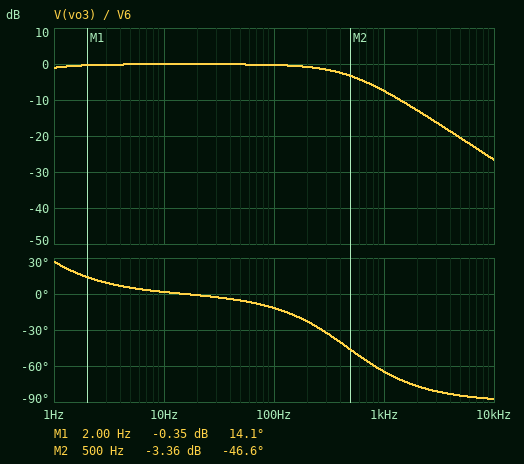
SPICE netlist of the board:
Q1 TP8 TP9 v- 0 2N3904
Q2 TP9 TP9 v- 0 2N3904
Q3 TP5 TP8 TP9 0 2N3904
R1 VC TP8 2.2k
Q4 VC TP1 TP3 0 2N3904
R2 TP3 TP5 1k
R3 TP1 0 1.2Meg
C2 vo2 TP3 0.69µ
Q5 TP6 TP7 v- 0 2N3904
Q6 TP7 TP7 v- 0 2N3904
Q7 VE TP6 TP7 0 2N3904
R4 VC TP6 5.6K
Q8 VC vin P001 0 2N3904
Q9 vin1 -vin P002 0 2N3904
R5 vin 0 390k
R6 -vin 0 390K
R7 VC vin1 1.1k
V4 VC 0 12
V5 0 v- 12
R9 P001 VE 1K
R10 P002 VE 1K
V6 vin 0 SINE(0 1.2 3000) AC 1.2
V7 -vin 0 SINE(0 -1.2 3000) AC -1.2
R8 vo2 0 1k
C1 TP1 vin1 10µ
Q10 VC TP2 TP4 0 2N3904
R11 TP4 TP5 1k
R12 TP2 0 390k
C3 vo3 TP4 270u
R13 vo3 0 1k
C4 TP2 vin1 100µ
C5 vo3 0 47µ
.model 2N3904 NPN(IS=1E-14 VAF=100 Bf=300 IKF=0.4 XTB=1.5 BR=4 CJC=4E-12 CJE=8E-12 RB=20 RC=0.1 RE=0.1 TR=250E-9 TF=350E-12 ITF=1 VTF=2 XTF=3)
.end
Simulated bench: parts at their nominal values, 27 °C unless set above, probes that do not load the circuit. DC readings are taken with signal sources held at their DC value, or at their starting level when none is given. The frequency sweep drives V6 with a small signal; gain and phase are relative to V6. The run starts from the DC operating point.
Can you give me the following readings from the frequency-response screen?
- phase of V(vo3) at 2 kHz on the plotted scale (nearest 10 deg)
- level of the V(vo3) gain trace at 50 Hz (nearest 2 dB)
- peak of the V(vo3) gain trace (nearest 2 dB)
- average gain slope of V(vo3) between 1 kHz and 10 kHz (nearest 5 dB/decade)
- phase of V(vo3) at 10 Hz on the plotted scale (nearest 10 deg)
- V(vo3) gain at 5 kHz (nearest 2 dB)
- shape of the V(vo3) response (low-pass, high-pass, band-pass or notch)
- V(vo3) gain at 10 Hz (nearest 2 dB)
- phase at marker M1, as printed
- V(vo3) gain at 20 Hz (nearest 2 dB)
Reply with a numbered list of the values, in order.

1. -80 deg
2. 0 dB
3. 0 dB
4. -20 dB/decade
5. 0 deg
6. -20 dB
7. low-pass
8. 0 dB
9. 14.1 deg
10. 0 dB
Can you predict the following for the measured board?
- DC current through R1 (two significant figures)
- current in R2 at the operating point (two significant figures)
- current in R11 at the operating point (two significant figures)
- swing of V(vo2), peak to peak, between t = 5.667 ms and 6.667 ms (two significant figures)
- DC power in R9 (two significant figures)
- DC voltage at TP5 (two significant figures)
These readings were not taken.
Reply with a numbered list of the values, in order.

1. 10 mA
2. 2.4 mA
3. 5.0 mA
4. 2.3 V
5. 4.0 mW
6. -11 V
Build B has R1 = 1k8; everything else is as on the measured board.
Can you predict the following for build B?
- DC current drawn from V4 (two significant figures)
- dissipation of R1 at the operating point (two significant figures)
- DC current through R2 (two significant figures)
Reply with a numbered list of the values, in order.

1. 28 mA
2. 280 mW
3. 2.4 mA
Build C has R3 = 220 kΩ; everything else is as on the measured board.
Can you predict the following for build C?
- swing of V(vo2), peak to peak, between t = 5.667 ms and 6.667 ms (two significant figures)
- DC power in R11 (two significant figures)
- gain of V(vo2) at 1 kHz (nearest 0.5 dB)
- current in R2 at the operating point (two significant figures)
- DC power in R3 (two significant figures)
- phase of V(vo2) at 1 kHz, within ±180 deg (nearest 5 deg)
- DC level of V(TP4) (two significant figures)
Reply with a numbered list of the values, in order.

1. 2.4 V
2. 20 mW
3. -1.5 dB
4. 5.7 mA
5. 61 µW
6. 5 deg
7. -5.7 V
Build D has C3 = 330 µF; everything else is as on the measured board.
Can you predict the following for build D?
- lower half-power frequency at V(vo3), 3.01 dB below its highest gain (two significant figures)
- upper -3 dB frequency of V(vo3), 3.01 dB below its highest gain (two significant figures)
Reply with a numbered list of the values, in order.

1. 420 mHz
2. 460 Hz
